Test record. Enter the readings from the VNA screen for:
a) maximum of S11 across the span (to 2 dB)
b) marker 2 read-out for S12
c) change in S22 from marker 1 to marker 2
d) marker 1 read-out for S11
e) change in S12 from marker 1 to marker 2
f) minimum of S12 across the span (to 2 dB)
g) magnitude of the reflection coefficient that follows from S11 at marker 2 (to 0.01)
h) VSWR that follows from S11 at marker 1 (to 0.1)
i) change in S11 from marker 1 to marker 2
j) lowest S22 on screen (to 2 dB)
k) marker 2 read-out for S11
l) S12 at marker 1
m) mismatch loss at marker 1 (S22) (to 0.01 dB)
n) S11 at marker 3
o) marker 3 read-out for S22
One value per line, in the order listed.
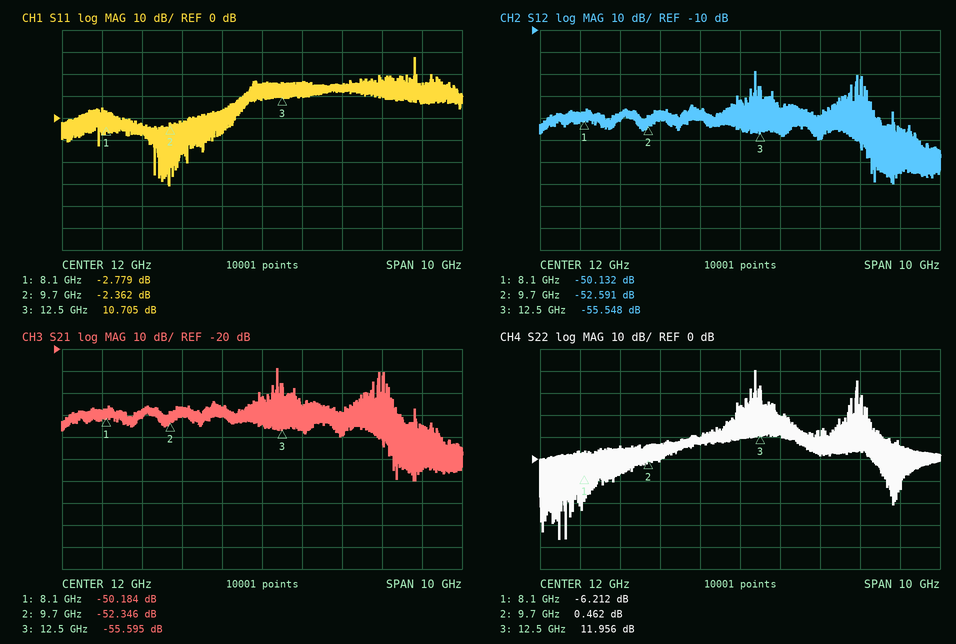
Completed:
28 dB
-52.591 dB
6.674 dB
-2.779 dB
-2.459 dB
-80 dB
0.76
6.3
0.417 dB
-36 dB
-2.362 dB
-50.132 dB
1.19 dB
10.705 dB
11.956 dB
